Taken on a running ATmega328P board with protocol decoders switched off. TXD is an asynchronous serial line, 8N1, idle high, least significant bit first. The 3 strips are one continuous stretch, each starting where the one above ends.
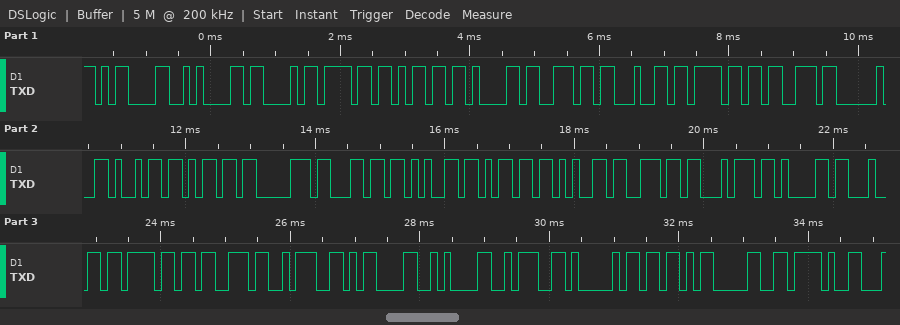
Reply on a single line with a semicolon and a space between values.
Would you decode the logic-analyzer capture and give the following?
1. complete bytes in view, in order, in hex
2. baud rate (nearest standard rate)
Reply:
0D 0A 43 6F 6D 61 6E 64 6F 73 20 69 6D 70 6C 65 6D 65 6E 74 61 64 6F 73 3A 0D 0A 3A 41 5B 30 2F; 9600 baud
